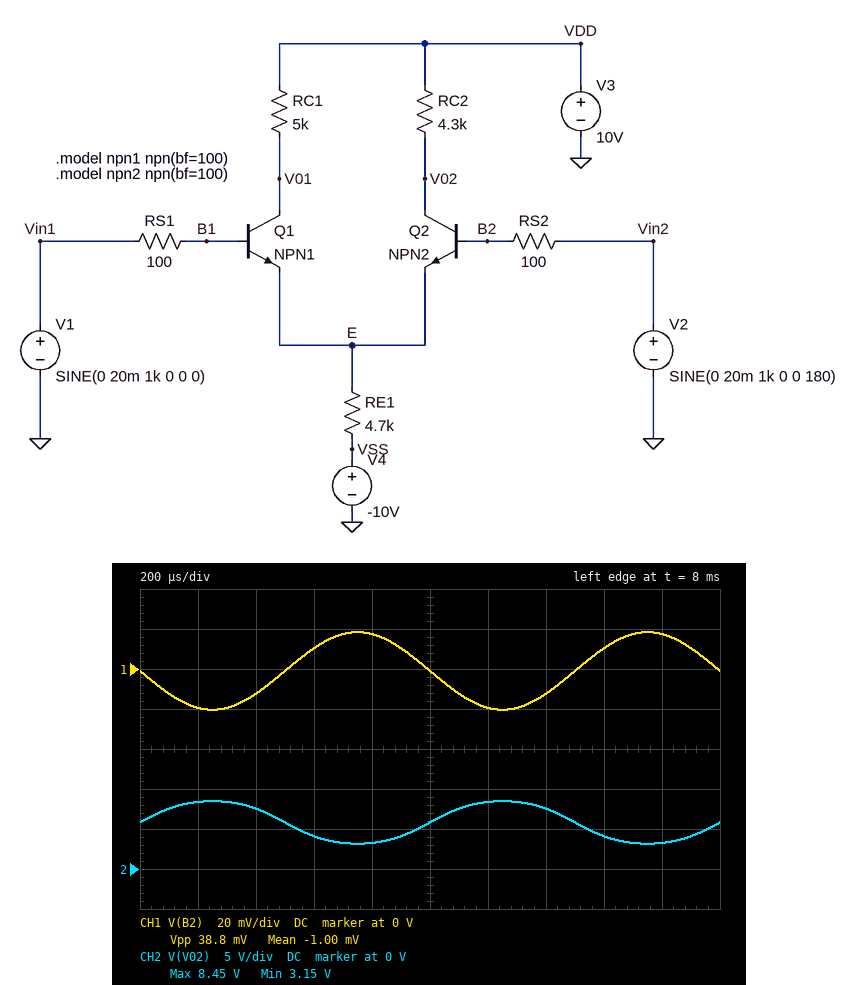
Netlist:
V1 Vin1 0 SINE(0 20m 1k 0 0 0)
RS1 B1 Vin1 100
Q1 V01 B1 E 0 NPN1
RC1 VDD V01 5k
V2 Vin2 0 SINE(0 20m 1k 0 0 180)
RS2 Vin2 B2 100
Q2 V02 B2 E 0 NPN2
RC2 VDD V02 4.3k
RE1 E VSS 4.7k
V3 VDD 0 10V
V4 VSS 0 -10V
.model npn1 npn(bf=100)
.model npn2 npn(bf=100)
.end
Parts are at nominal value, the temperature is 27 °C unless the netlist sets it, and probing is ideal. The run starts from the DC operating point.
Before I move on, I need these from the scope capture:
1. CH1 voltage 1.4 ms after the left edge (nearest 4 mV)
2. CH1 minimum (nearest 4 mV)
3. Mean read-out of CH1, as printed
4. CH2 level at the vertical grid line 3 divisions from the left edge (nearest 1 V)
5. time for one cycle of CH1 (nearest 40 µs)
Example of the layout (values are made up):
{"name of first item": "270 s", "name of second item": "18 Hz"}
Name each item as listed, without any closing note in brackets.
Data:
{"CH1 voltage 1.4 ms after the left edge": "-12 mV", "CH1 minimum": "-20 mV", "Mean read-out of CH1, as printed": "-1.00 mV", "CH2 level at the vertical grid line 3 divisions from the left edge": "4 V", "time for one cycle of CH1": "1.00 ms"}
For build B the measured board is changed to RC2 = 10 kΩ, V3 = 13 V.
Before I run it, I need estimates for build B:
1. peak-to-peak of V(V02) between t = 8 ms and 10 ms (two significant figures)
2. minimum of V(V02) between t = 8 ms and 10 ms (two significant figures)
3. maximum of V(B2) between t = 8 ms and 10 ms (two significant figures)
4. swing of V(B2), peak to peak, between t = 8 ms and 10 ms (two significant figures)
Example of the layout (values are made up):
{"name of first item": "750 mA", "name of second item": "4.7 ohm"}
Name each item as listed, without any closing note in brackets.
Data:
{"peak-to-peak of V(V02) between t = 8 ms and 10 ms": "10 V", "minimum of V(V02) between t = 8 ms and 10 ms": "-700 mV", "maximum of V(B2) between t = 8 ms and 10 ms": "10 mV", "swing of V(B2), peak to peak, between t = 8 ms and 10 ms": "30 mV"}
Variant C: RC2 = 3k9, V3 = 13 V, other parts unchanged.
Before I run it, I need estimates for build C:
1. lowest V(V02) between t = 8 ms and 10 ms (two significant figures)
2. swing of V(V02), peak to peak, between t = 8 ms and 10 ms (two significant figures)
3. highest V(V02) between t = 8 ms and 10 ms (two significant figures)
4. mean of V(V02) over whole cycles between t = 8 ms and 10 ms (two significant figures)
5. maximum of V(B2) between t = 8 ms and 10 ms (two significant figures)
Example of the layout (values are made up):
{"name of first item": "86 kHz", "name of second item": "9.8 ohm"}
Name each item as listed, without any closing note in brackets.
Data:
{"lowest V(V02) between t = 8 ms and 10 ms": "6.8 V", "swing of V(V02), peak to peak, between t = 8 ms and 10 ms": "4.8 V", "highest V(V02) between t = 8 ms and 10 ms": "12 V", "mean of V(V02) over whole cycles between t = 8 ms and 10 ms": "9.2 V", "maximum of V(B2) between t = 8 ms and 10 ms": "18 mV"}
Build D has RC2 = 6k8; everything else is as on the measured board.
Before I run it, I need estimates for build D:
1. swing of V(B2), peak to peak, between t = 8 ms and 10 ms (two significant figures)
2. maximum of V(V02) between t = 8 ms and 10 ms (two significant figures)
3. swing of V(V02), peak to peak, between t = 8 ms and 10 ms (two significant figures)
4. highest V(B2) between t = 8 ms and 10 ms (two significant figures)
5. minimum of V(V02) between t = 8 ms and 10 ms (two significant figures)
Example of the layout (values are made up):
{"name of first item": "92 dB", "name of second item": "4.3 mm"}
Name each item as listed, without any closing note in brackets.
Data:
{"swing of V(B2), peak to peak, between t = 8 ms and 10 ms": "38 mV", "maximum of V(V02) between t = 8 ms and 10 ms": "7.6 V", "swing of V(V02), peak to peak, between t = 8 ms and 10 ms": "8.2 V", "highest V(B2) between t = 8 ms and 10 ms": "17 mV", "minimum of V(V02) between t = 8 ms and 10 ms": "-640 mV"}
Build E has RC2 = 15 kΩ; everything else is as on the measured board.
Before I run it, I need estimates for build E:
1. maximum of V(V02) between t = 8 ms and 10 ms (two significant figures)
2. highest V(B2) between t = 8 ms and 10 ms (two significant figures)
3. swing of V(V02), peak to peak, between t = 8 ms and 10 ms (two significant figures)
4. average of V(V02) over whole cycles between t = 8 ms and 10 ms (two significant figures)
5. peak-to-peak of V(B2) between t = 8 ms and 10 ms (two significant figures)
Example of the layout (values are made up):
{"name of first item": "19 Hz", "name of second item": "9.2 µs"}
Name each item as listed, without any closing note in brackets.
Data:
{"maximum of V(V02) between t = 8 ms and 10 ms": "4.7 V", "highest V(B2) between t = 8 ms and 10 ms": "-8.1 mV", "swing of V(V02), peak to peak, between t = 8 ms and 10 ms": "5.4 V", "average of V(V02) over whole cycles between t = 8 ms and 10 ms": "670 mV", "peak-to-peak of V(B2) between t = 8 ms and 10 ms": "12 mV"}
